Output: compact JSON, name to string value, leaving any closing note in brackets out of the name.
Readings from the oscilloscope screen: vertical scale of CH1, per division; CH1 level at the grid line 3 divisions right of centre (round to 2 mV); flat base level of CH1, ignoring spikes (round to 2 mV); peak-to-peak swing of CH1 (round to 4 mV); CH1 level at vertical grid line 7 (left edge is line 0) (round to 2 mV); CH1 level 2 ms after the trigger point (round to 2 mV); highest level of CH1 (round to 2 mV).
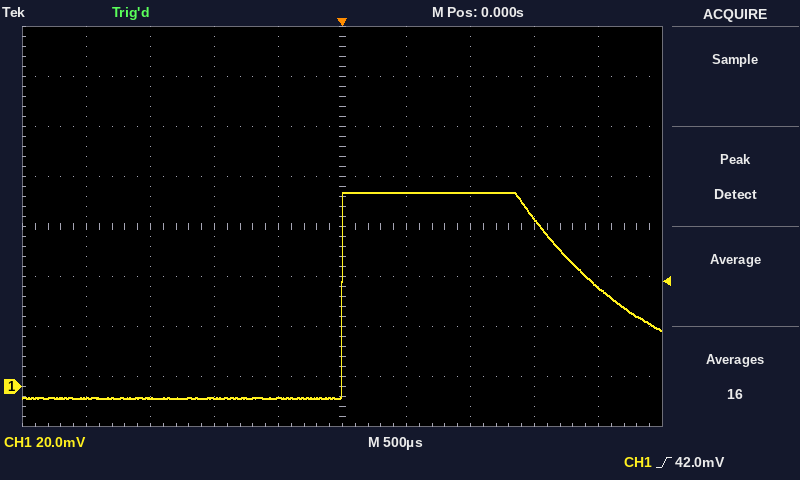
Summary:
{"vertical scale of CH1, per division": "20 mV", "CH1 level at the grid line 3 divisions right of centre": "68 mV", "flat base level of CH1, ignoring spikes": "-4 mV", "peak-to-peak swing of CH1": "84 mV", "CH1 level at vertical grid line 7 (left edge is line 0)": "78 mV", "CH1 level 2 ms after the trigger point": "40 mV", "highest level of CH1": "78 mV"}
